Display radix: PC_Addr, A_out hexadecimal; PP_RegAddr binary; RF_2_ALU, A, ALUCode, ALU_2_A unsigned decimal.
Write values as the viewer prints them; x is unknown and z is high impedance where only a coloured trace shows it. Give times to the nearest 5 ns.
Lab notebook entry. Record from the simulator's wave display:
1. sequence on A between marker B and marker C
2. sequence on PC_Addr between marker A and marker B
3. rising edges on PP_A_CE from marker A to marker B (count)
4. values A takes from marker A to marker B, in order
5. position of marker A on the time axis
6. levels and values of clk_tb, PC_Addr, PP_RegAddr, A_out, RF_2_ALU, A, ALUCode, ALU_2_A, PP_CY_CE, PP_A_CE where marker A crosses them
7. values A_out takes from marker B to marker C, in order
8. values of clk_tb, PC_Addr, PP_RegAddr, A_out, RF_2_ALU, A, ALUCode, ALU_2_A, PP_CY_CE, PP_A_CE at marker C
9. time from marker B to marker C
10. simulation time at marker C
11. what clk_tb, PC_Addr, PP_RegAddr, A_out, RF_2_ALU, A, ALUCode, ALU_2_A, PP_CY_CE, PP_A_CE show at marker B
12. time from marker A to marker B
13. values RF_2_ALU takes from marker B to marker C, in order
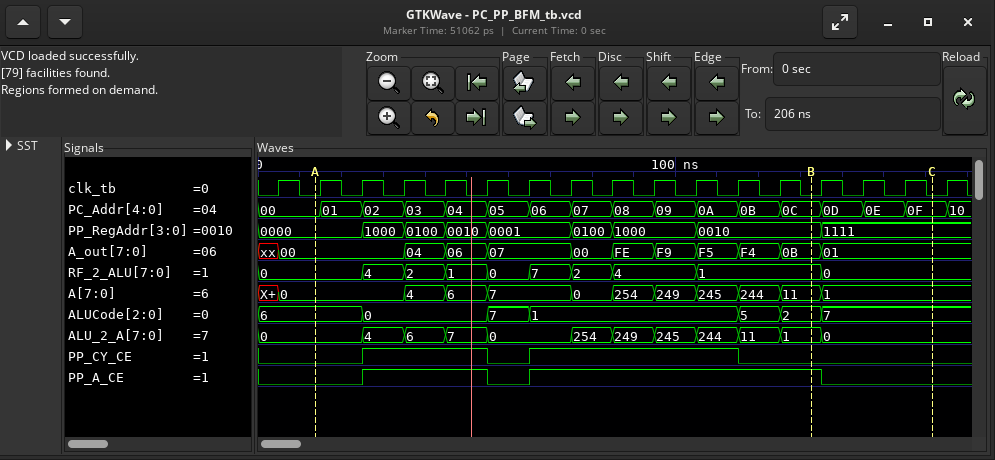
11, 1
00, 01, 02, 03, 04, 05, 06, 07, 08, 09, 0A, 0B, 0C
2
0, 4, 6, 7, 0, 254, 249, 245, 244, 11
15 ns
clk_tb=0, PC_Addr=00, PP_RegAddr=0000, A_out=00, RF_2_ALU=0, A=0, ALUCode=6, ALU_2_A=0, PP_CY_CE=0, PP_A_CE=0
0B, 01
clk_tb=0, PC_Addr=0F, PP_RegAddr=1111, A_out=01, RF_2_ALU=0, A=1, ALUCode=7, ALU_2_A=0, PP_CY_CE=0, PP_A_CE=0
30 ns
160 ns
clk_tb=0, PC_Addr=0C, PP_RegAddr=0010, A_out=0B, RF_2_ALU=1, A=11, ALUCode=2, ALU_2_A=1, PP_CY_CE=0, PP_A_CE=1
120 ns
1, 0
